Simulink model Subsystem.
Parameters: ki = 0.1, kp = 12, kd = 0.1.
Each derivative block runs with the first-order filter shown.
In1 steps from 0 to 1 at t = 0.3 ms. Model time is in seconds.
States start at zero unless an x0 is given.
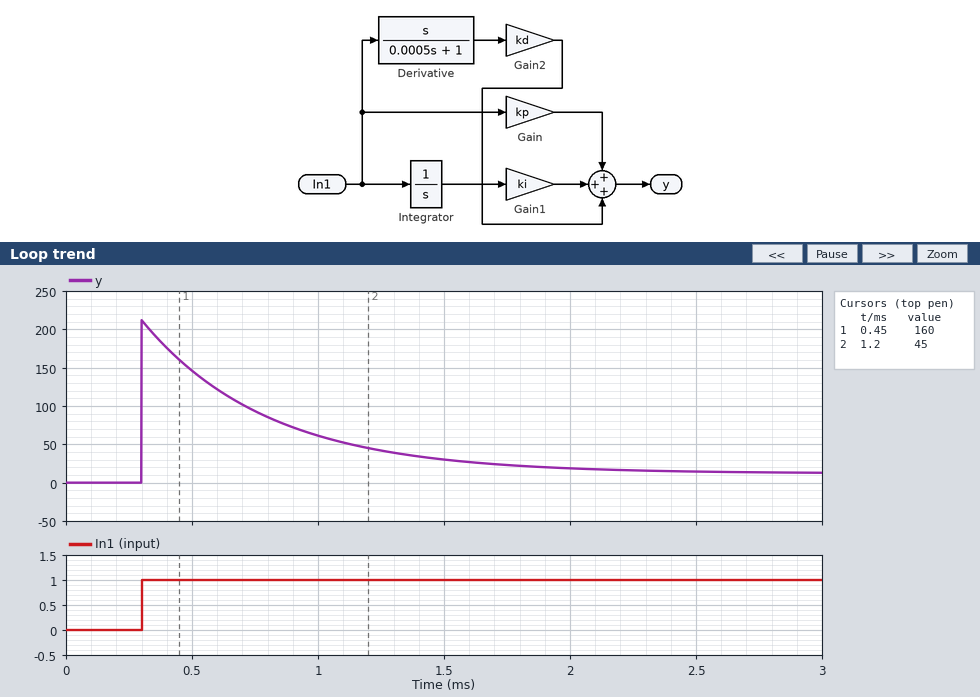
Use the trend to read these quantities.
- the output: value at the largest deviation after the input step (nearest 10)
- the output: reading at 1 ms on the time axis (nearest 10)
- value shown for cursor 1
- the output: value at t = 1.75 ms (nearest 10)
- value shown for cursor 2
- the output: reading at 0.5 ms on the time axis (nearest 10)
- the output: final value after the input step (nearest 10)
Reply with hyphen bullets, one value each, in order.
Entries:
- 210
- 60
- 160
- 20
- 45
- 150
- 10
